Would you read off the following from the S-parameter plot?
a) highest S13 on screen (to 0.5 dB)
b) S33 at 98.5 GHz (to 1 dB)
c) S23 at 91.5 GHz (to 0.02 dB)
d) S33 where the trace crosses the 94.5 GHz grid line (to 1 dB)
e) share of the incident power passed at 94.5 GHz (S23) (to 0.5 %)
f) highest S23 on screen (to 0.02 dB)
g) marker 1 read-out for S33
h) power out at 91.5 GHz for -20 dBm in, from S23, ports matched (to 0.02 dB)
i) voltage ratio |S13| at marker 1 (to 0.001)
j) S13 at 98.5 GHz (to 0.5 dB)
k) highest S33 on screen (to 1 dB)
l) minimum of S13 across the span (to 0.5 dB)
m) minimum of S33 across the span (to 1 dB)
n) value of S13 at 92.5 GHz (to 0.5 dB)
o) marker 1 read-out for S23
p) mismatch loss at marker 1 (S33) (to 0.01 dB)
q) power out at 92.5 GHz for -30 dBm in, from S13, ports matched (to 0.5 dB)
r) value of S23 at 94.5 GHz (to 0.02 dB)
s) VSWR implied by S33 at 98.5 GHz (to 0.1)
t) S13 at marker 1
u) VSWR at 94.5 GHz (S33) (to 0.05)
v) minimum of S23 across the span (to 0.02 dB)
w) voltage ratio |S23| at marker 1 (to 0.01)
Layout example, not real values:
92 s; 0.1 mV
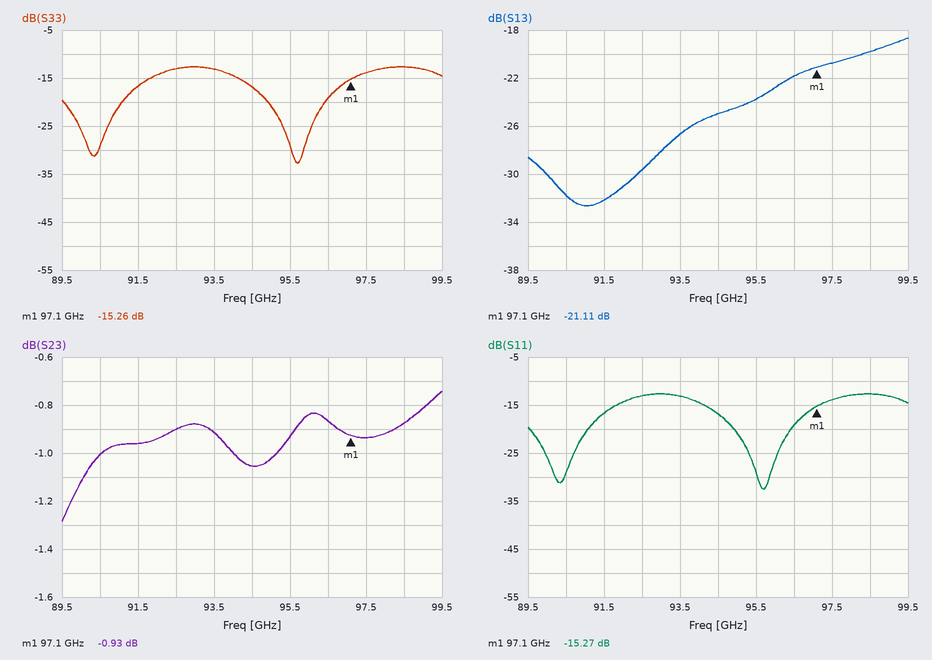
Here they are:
-18.5 dB; -13 dB; -0.96 dB; -17 dB; 78.5 %; -0.74 dB; -15.26 dB; -20.96 dBm; 0.088; -20.0 dB; -13 dB; -32.5 dB; -33 dB; -29.5 dB; -0.93 dB; 0.13 dB; -59.5 dBm; -1.06 dB; 1.6; -21.11 dB; 1.35; -1.28 dB; 0.90
